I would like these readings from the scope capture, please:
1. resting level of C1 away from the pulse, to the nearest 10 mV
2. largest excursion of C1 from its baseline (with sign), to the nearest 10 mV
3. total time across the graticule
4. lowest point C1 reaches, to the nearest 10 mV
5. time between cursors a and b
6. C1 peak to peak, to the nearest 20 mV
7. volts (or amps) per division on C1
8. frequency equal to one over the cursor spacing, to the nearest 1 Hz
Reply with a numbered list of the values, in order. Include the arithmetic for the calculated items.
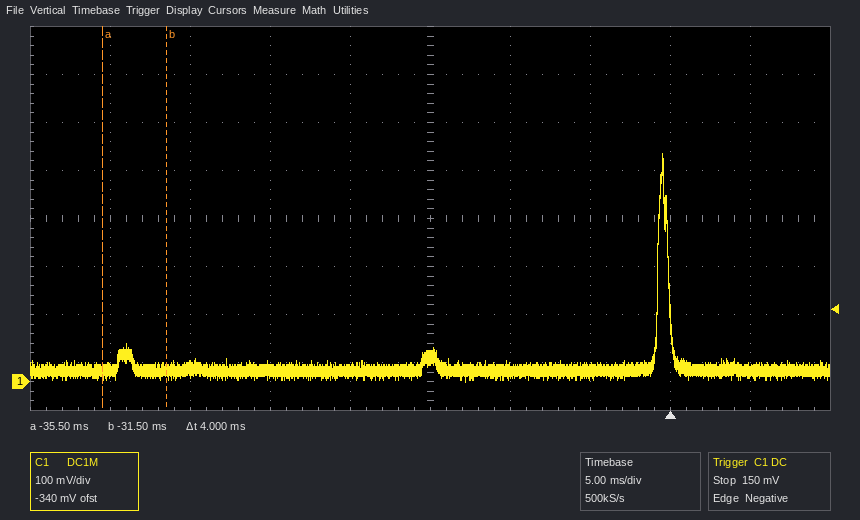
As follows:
1. 20 mV
2. +450 mV
3. 50 ms
4. 0 mV
5. 4 ms
6. 480 mV
7. 100 mV
8. 1 / 4 ms ≈ 250 Hz
